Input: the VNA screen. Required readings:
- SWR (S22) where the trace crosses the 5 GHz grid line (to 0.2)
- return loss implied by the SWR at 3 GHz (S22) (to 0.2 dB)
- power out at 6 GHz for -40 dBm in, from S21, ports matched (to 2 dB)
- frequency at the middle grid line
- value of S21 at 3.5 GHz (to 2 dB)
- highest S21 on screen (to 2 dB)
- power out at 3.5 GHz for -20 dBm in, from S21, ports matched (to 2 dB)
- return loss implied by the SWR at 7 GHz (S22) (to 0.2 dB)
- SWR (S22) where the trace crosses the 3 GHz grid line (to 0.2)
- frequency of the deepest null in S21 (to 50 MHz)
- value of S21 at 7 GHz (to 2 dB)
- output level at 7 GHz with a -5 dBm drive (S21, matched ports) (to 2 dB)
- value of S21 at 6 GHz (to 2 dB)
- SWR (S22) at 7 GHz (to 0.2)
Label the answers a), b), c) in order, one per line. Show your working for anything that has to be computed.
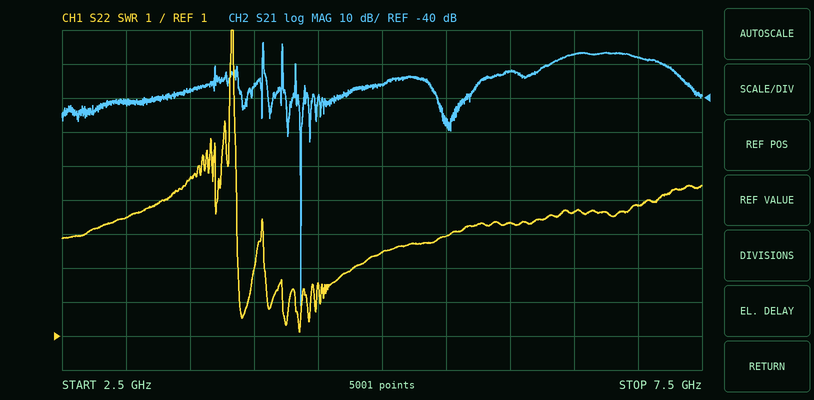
a) 3.4
b) −20 log10((4.4 − 1)/(4.4 + 1)) ≈ 4.0 dB
c) -40 dBm + (-32 dB) = -72 dBm
d) 5 GHz
e) -38 dB
f) -24 dB
g) -20 dBm + (-38 dB) = -58 dBm
h) −20 log10((4.8 − 1)/(4.8 + 1)) ≈ 3.67 dB, so 3.6 dB to the nearest 0.2 dB
i) 4.4
j) 4.35 GHz
k) -28 dB
l) -5 dBm + (-28 dB) = -34 dBm
m) -32 dB
n) 4.8
